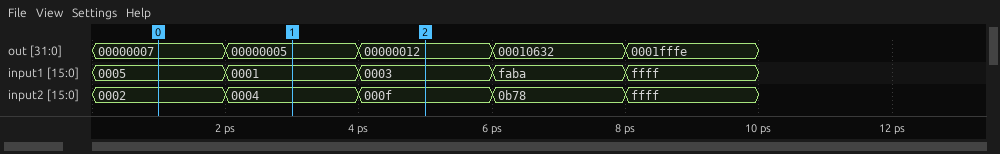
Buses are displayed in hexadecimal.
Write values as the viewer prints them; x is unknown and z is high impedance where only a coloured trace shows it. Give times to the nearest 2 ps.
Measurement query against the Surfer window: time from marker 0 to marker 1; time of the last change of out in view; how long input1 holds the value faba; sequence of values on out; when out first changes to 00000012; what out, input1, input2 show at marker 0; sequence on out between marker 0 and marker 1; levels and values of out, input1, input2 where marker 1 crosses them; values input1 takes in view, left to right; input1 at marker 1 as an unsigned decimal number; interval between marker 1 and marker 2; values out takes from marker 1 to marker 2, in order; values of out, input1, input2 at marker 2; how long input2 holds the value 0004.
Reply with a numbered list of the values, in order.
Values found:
1. 2 ps
2. 8 ps
3. 2 ps
4. 00000007, 00000005, 00000012, 00010632, 0001fffe
5. 4 ps
6. out=00000007, input1=0005, input2=0002
7. 00000007, 00000005
8. out=00000005, input1=0001, input2=0004
9. 0005, 0001, 0003, faba, ffff
10. 1
11. 2 ps
12. 00000005, 00000012
13. out=00000012, input1=0003, input2=000f
14. 2 ps
